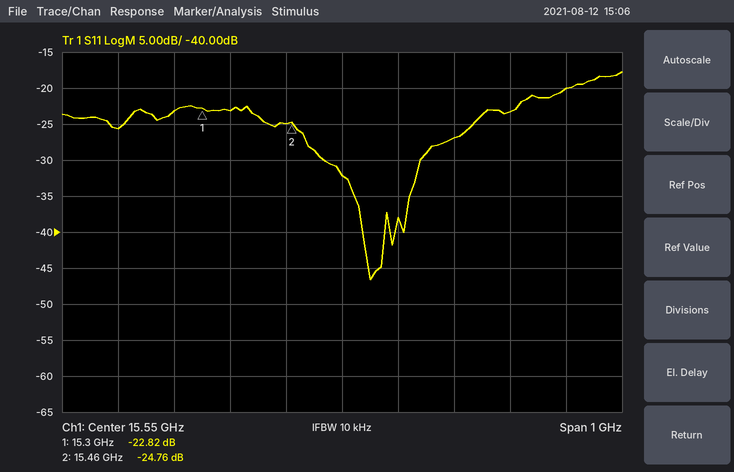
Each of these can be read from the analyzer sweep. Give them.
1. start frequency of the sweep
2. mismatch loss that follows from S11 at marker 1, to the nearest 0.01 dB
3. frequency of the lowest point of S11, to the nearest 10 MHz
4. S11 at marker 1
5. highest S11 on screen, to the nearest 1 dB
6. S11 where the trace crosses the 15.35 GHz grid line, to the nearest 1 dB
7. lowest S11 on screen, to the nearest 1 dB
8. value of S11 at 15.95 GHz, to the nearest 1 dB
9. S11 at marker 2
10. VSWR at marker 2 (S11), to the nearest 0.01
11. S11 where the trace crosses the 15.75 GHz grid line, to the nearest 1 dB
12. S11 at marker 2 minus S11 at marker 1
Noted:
15.05 GHz
0.02 dB
15.60 GHz
-22.82 dB
-18 dB
-23 dB
-47 dB
-20 dB
-24.76 dB
1.12
-27 dB
-1.94 dB
